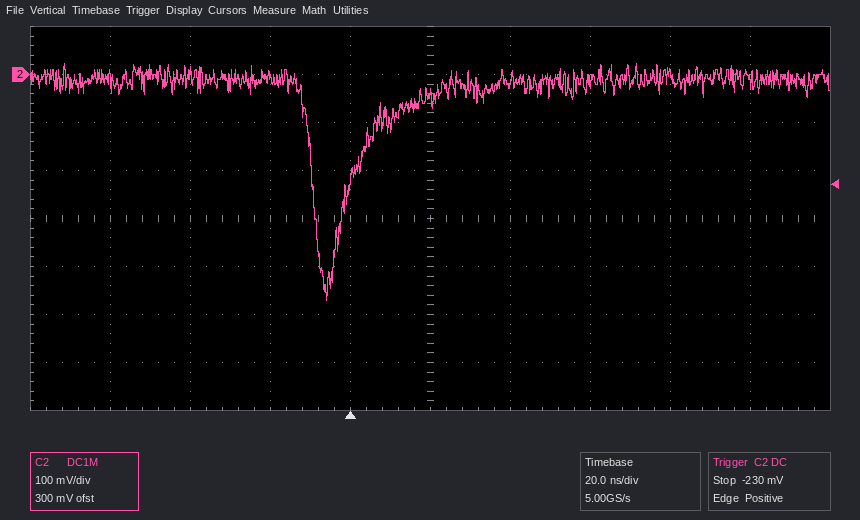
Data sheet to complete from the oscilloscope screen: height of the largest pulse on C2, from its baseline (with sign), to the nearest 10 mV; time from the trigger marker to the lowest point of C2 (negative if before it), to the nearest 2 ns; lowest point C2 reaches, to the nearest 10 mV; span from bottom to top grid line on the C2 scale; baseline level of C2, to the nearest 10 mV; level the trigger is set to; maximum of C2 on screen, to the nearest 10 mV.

-460 mV
-6 ns
-470 mV
800 mV
-10 mV
-230 mV
20 mV
